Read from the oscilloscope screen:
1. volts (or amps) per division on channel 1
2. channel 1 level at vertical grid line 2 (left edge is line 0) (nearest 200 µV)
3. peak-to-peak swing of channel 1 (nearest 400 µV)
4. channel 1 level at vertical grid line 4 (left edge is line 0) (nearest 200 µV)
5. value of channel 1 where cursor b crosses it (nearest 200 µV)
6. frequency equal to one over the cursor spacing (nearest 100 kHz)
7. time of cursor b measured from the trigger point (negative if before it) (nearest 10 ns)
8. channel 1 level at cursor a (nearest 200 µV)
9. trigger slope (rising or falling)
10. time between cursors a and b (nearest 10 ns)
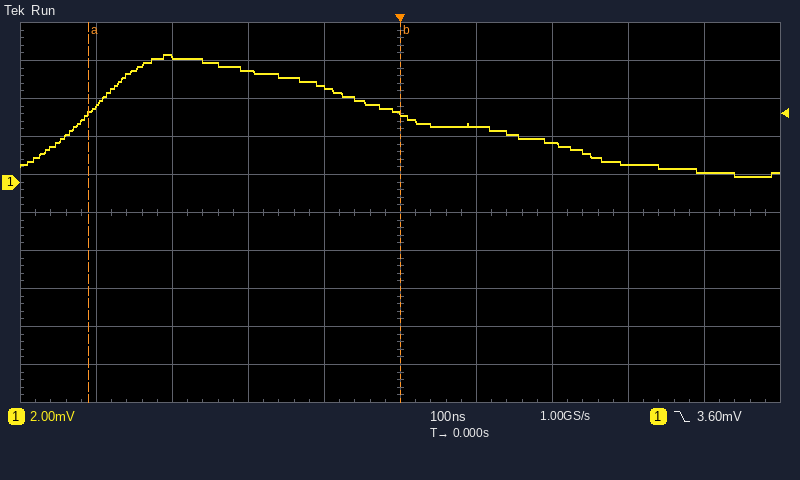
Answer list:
2 mV
6.6 mV
6.4 mV
5.0 mV
3.6 mV
2.4 MHz
0 ns
3.6 mV
falling
410 ns
